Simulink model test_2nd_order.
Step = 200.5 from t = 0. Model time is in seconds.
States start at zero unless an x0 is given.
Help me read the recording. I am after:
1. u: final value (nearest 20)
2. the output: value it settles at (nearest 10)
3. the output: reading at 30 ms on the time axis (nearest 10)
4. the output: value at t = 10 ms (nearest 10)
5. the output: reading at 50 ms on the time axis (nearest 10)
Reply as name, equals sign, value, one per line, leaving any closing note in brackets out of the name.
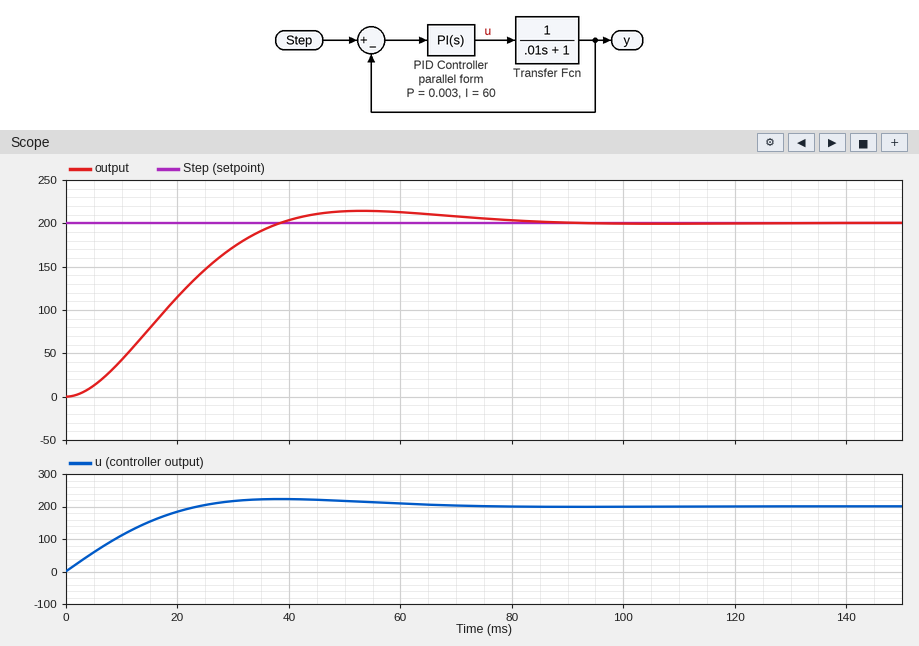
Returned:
u: final value = 200
the output: value it settles at = 200
the output: reading at 30 ms on the time axis = 170
the output: value at t = 10 ms = 40
the output: reading at 50 ms on the time axis = 210
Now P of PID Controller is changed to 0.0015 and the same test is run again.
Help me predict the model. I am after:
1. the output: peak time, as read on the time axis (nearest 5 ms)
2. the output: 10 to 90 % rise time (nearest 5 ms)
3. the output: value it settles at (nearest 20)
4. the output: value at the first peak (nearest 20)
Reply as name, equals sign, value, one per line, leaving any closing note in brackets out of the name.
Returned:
the output: peak time, as read on the time axis = 55 ms
the output: 10 to 90 % rise time = 25 ms
the output: value it settles at = 200
the output: value at the first peak = 220
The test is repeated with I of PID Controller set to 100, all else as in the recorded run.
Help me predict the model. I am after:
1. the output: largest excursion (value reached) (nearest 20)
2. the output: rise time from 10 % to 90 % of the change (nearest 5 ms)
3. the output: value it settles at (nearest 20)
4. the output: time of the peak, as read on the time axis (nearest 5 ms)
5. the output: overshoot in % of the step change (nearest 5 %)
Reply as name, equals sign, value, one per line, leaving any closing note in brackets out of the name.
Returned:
the output: largest excursion (value reached) = 240
the output: rise time from 10 % to 90 % of the change = 15 ms
the output: value it settles at = 200
the output: time of the peak, as read on the time axis = 35 ms
the output: overshoot in % of the step change = 15 %
